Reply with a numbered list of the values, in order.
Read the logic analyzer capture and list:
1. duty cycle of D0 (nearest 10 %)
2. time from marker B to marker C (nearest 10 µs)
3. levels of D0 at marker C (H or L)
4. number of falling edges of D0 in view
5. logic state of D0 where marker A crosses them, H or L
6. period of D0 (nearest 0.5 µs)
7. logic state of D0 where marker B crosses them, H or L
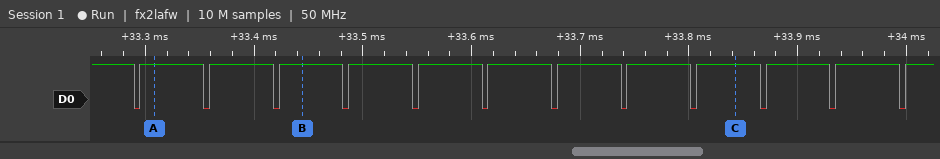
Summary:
1. 90 %
2. 400 µs
3. D0=H
4. 12
5. D0=H
6. 64 µs
7. D0=H
